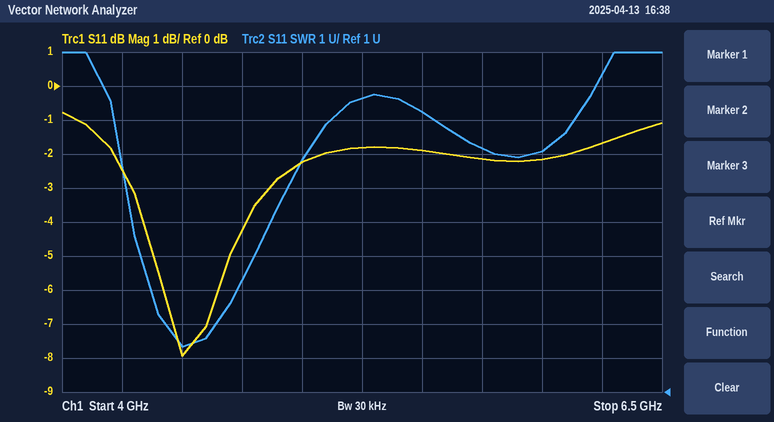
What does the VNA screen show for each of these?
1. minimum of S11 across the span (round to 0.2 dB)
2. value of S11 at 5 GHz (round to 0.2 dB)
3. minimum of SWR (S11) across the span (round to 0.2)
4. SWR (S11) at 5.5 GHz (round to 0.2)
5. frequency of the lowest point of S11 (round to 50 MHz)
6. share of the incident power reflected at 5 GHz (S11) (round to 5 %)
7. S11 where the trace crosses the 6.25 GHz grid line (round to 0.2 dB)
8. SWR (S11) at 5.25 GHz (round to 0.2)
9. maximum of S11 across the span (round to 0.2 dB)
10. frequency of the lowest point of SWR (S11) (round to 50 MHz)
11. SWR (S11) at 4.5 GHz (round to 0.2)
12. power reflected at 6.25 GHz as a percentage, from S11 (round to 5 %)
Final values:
-8.0 dB
-2.2 dB
2.4
9.2
4.50 GHz
60 %
-1.6 dB
9.6
-0.8 dB
4.50 GHz
2.4
70 %
